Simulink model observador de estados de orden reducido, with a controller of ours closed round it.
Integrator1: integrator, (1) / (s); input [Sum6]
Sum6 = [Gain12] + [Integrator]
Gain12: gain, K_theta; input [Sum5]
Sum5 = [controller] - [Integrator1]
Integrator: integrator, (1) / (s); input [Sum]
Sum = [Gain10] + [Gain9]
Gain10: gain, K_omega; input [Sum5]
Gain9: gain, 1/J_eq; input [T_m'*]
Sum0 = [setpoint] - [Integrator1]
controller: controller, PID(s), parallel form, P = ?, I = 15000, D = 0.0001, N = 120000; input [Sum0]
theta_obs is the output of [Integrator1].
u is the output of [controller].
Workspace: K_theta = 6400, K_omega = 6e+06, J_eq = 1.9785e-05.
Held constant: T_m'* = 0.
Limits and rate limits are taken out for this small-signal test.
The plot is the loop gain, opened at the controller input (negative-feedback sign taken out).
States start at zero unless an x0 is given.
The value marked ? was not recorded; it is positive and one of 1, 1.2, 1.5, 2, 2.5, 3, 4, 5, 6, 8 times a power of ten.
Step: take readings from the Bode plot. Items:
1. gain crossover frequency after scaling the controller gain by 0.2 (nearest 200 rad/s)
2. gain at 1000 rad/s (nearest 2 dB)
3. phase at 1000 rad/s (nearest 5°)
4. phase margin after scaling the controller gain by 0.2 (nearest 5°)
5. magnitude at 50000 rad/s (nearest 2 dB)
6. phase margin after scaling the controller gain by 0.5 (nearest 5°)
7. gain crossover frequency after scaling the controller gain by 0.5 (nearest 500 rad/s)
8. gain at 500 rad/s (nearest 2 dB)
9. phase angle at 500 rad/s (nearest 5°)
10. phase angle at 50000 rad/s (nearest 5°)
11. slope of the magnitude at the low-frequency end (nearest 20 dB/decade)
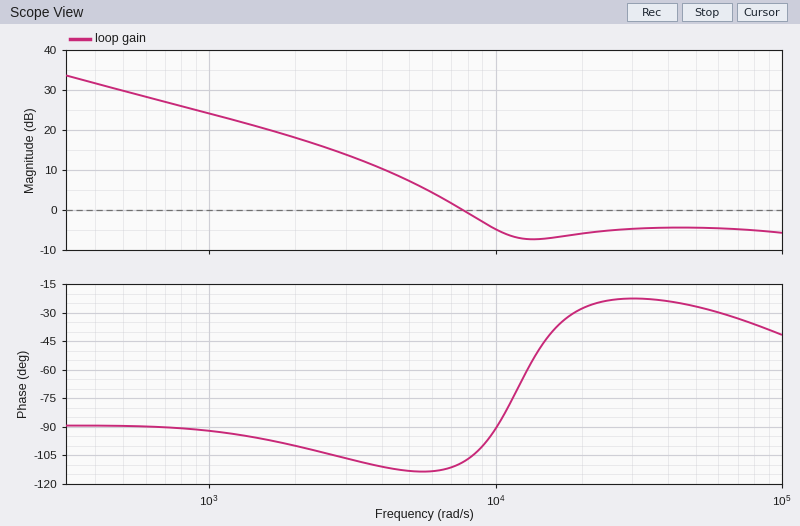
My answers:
3000 rad/s
24 dB
-90°
75°
-4 dB
65°
5500 rad/s
30 dB
-90°
-25°
-20 dB/decade
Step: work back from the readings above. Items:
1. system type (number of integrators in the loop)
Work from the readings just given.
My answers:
1
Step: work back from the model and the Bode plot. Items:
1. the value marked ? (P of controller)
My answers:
0.8
